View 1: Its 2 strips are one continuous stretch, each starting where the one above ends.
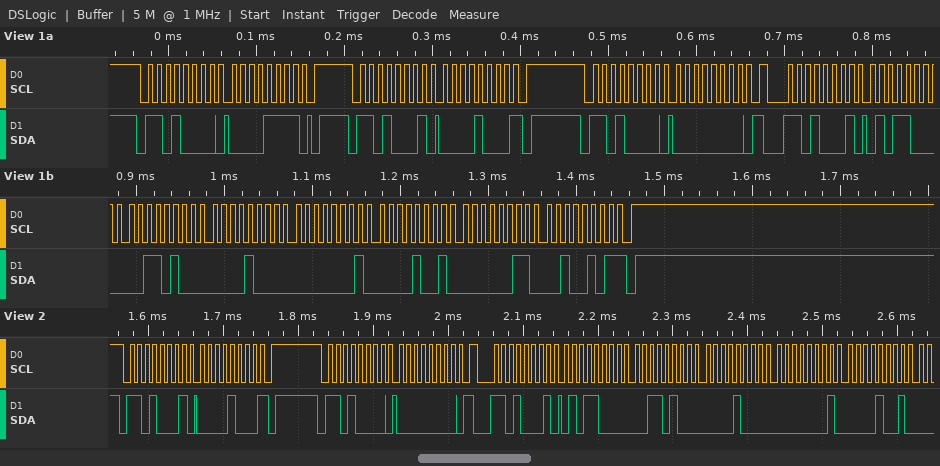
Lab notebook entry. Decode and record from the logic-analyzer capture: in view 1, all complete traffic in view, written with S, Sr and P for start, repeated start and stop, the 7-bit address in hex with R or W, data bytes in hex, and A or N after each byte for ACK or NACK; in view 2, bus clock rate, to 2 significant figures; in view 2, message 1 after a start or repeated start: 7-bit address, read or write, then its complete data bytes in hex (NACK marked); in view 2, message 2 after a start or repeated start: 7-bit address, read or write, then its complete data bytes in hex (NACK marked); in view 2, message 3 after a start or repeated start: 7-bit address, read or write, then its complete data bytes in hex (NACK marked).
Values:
S 68W A 0F A P S 68R A 08 N P S 68W A 00 A Sr 68R A 58 A 34 A 08 A 01 A 09 A 03 A 25 N P
100 kHz
0x68 read: 08 NACK
0x68 write: 00
0x68 read: 58 34 08 01 09
